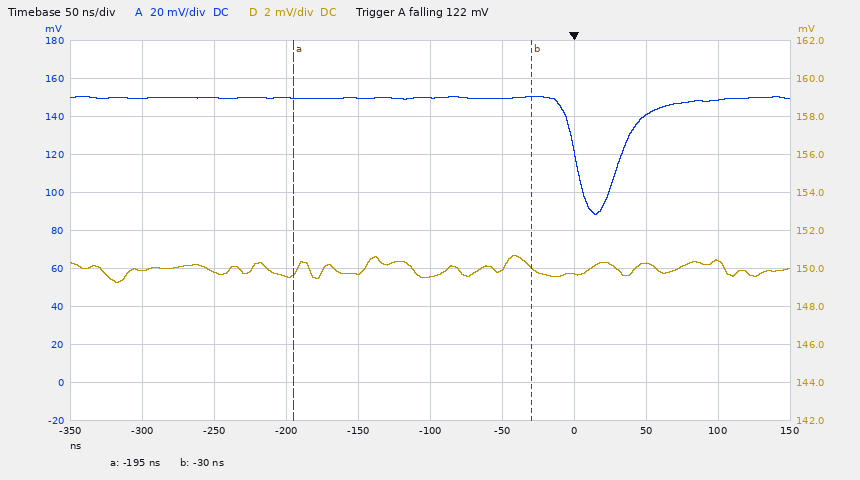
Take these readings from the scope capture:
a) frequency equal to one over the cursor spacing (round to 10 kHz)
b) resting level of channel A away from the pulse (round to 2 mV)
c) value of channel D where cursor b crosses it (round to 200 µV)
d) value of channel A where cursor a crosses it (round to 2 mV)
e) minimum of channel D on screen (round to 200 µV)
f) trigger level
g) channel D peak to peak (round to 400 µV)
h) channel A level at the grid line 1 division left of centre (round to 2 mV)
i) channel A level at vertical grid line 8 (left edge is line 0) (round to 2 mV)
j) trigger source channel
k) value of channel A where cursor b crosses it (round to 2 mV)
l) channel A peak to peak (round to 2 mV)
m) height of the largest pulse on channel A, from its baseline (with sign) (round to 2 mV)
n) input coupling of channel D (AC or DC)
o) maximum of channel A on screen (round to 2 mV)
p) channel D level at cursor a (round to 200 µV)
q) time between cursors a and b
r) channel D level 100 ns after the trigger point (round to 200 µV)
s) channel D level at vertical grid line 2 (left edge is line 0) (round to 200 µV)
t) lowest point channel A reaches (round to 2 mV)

6.06 MHz
150 mV
150.0 mV
150 mV
149.2 mV
122 mV
1.6 mV
150 mV
140 mV
channel A
150 mV
62 mV
-62 mV
DC
150 mV
149.8 mV
165 ns
150.4 mV
149.8 mV
88 mV
